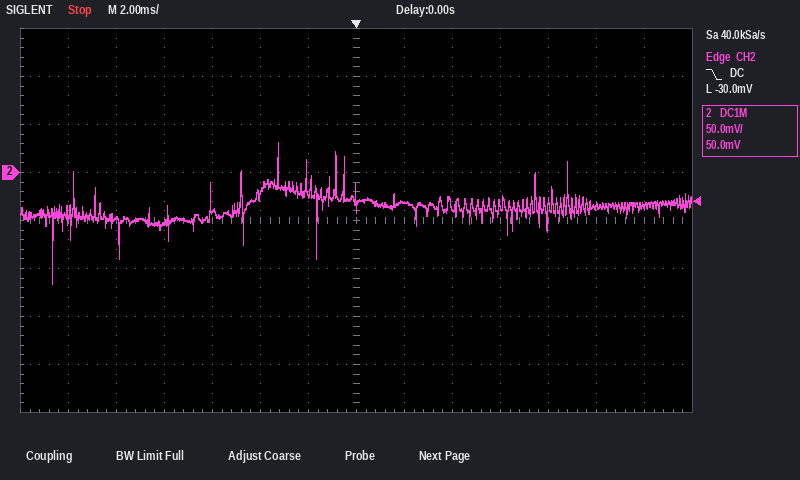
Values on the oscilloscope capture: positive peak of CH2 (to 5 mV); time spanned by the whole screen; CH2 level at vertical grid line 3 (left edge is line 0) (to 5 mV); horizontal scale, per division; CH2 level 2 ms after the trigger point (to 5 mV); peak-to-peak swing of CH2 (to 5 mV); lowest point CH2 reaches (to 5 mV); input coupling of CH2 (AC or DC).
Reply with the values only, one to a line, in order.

30 mV
28 ms
-50 mV
2 ms
-30 mV
145 mV
-115 mV
DC
